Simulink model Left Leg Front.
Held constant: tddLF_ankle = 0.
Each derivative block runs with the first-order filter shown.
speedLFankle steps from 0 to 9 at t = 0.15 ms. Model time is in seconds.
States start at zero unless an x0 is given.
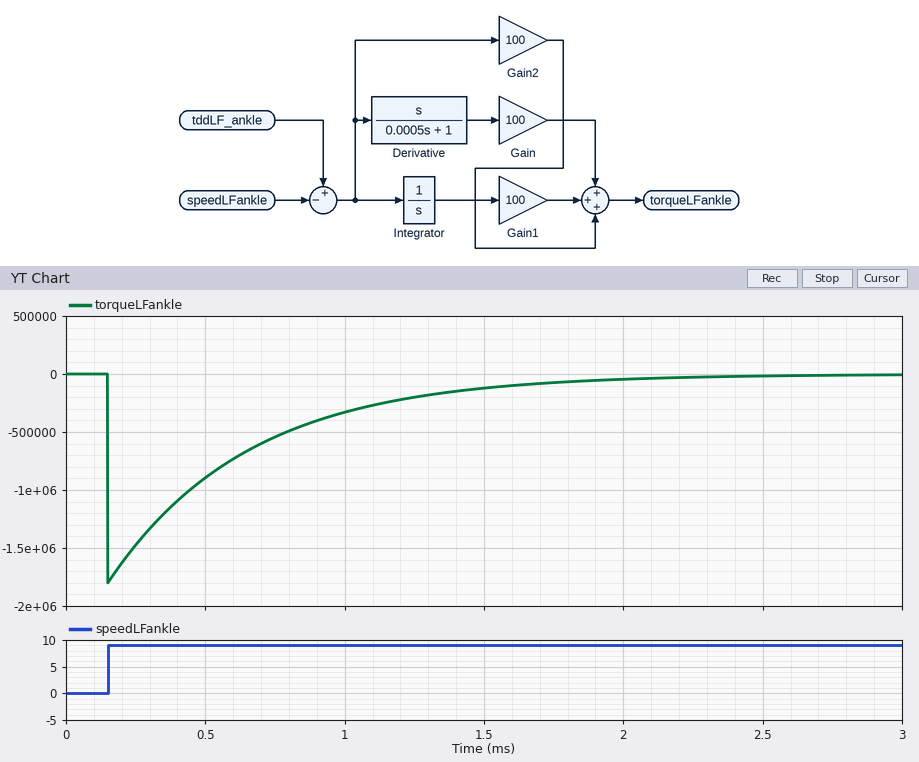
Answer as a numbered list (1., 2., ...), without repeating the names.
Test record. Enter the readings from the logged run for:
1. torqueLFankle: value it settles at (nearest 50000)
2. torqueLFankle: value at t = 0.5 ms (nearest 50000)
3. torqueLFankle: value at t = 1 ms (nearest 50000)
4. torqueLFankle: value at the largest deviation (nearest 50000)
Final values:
1. 0
2. -900000
3. -350000
4. -1800000
